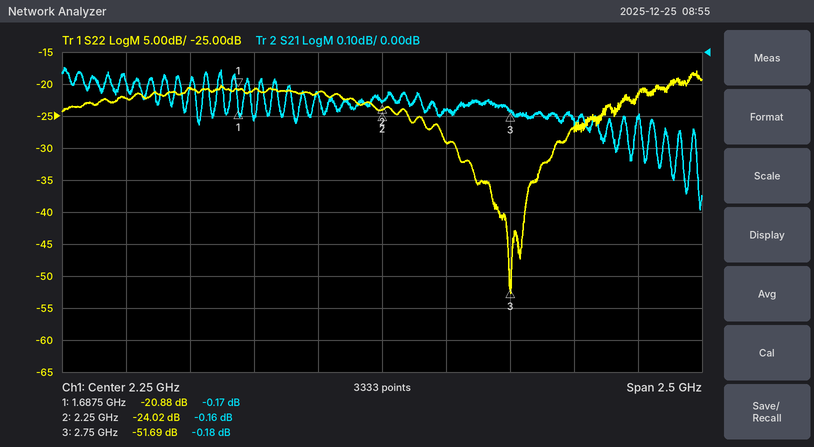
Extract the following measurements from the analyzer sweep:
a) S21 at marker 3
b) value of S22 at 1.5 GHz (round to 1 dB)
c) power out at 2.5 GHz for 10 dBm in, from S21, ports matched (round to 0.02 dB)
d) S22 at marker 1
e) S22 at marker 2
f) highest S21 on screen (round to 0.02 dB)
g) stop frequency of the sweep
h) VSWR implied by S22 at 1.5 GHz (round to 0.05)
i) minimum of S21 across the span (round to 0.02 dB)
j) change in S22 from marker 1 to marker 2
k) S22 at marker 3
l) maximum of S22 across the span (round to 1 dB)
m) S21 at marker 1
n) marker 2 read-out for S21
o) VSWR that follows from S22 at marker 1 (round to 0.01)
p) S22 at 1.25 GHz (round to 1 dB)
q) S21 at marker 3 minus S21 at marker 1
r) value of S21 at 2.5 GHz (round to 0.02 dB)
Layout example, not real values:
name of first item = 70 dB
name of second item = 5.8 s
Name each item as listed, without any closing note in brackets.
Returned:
S21 at marker 3 = -0.18 dB
value of S22 at 1.5 GHz = -21 dB
power out at 2.5 GHz for 10 dBm in, from S21, ports matched = 9.82 dBm
S22 at marker 1 = -20.88 dB
S22 at marker 2 = -24.02 dB
highest S21 on screen = -0.04 dB
stop frequency of the sweep = 3.5 GHz
VSWR implied by S22 at 1.5 GHz = 1.20
minimum of S21 across the span = -0.50 dB
change in S22 from marker 1 to marker 2 = -3.14 dB
S22 at marker 3 = -51.69 dB
maximum of S22 across the span = -18 dB
S21 at marker 1 = -0.17 dB
marker 2 read-out for S21 = -0.16 dB
VSWR that follows from S22 at marker 1 = 1.20
S22 at 1.25 GHz = -22 dB
S21 at marker 3 minus S21 at marker 1 = -0.01 dB
value of S21 at 2.5 GHz = -0.18 dB
